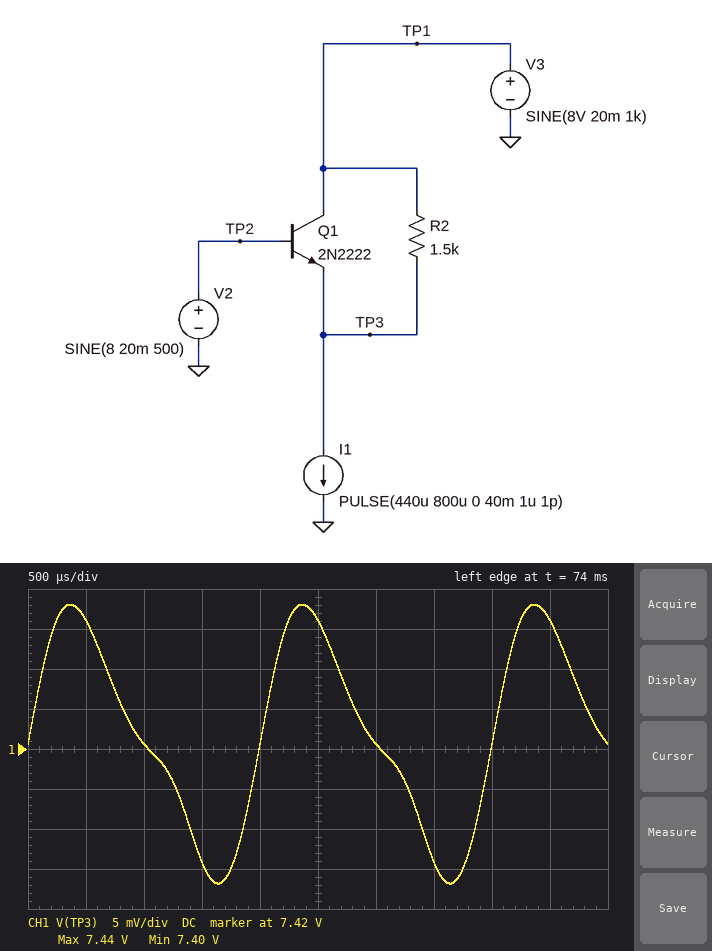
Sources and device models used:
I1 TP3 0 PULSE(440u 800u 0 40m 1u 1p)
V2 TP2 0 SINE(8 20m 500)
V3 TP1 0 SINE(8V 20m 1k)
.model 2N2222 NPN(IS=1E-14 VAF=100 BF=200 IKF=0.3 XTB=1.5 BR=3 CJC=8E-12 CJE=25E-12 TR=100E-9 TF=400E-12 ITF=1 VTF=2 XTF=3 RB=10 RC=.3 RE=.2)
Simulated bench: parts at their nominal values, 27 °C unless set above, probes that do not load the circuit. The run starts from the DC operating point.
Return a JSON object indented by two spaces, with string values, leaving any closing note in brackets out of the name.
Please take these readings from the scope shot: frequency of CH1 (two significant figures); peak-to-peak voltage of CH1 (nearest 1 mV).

{
  "frequency of CH1": "500 Hz",
  "peak-to-peak voltage of CH1": "35 mV"
}
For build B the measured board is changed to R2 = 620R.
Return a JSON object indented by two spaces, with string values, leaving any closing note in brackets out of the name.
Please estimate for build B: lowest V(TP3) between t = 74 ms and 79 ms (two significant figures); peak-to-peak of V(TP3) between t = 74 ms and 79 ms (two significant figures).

{
  "lowest V(TP3) between t = 74 ms and 79 ms": "7.7 V",
  "peak-to-peak of V(TP3) between t = 74 ms and 79 ms": "40 mV"
}
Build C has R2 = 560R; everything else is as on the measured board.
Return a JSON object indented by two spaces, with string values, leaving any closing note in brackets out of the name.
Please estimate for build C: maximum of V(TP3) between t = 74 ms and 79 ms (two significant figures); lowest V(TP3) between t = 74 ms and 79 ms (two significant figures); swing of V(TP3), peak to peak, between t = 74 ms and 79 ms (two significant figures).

{
  "maximum of V(TP3) between t = 74 ms and 79 ms": "7.8 V",
  "lowest V(TP3) between t = 74 ms and 79 ms": "7.7 V",
  "swing of V(TP3), peak to peak, between t = 74 ms and 79 ms": "40 mV"
}
